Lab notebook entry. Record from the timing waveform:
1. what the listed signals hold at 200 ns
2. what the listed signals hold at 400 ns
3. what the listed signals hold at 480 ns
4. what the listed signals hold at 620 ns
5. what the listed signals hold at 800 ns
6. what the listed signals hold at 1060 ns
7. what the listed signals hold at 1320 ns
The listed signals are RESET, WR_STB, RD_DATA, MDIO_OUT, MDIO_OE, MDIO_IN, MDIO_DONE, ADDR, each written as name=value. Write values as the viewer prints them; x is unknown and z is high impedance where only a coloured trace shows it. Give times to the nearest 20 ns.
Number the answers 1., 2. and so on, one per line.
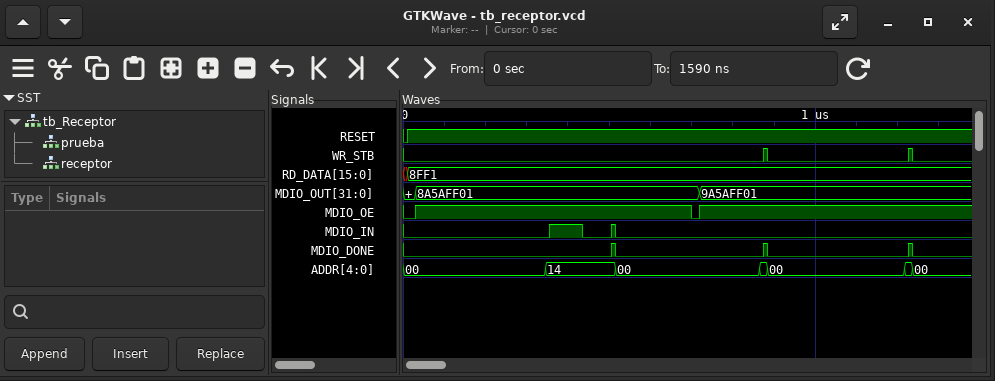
1. RESET=1, WR_STB=0, RD_DATA=8FF1, MDIO_OUT=8A5AFF01, MDIO_OE=1, MDIO_IN=0, MDIO_DONE=0, ADDR=00
2. RESET=1, WR_STB=0, RD_DATA=8FF1, MDIO_OUT=8A5AFF01, MDIO_OE=1, MDIO_IN=1, MDIO_DONE=0, ADDR=14
3. RESET=1, WR_STB=0, RD_DATA=8FF1, MDIO_OUT=8A5AFF01, MDIO_OE=1, MDIO_IN=0, MDIO_DONE=0, ADDR=14
4. RESET=1, WR_STB=0, RD_DATA=8FF1, MDIO_OUT=8A5AFF01, MDIO_OE=1, MDIO_IN=0, MDIO_DONE=0, ADDR=00
5. RESET=1, WR_STB=0, RD_DATA=8FF1, MDIO_OUT=9A5AFF01, MDIO_OE=1, MDIO_IN=0, MDIO_DONE=0, ADDR=00
6. RESET=1, WR_STB=0, RD_DATA=8FF1, MDIO_OUT=9A5AFF01, MDIO_OE=1, MDIO_IN=0, MDIO_DONE=0, ADDR=00
7. RESET=1, WR_STB=0, RD_DATA=8FF1, MDIO_OUT=9A5AFF01, MDIO_OE=1, MDIO_IN=0, MDIO_DONE=0, ADDR=00
